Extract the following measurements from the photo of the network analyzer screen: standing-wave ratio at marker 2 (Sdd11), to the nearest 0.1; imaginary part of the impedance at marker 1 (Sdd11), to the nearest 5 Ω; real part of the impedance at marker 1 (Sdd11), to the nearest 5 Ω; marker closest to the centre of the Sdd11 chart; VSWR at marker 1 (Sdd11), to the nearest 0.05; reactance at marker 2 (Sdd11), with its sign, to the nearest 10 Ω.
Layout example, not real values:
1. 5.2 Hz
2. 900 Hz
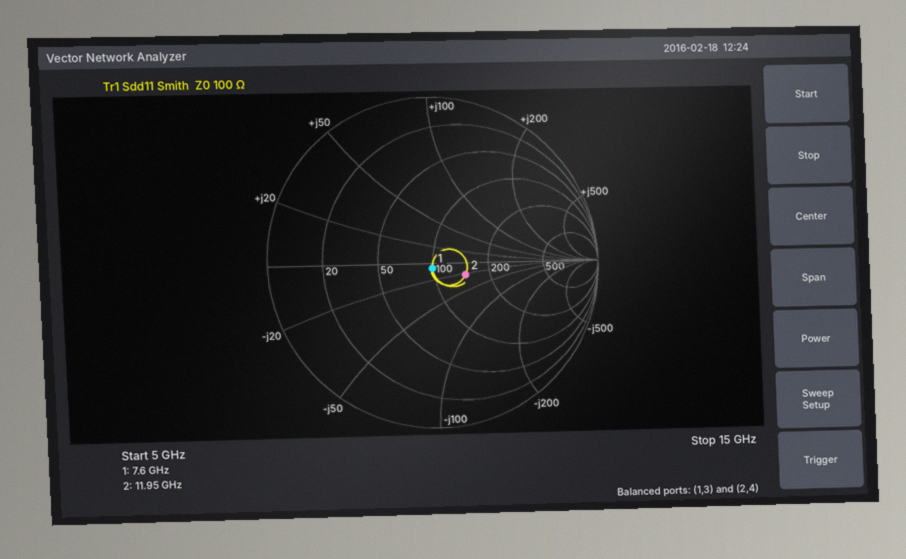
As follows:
1. 1.5
2. -5 Ω
3. 100 Ω
4. marker 1
5. 1.05
6. -20 Ω
